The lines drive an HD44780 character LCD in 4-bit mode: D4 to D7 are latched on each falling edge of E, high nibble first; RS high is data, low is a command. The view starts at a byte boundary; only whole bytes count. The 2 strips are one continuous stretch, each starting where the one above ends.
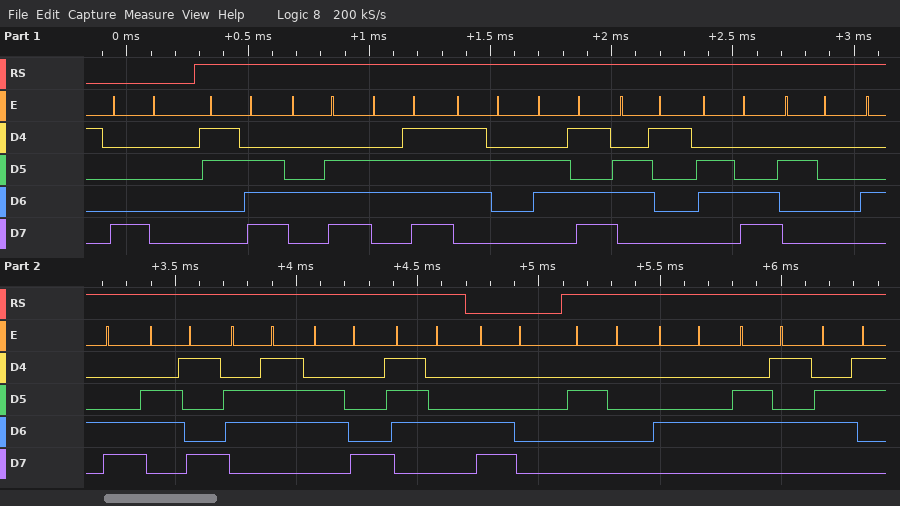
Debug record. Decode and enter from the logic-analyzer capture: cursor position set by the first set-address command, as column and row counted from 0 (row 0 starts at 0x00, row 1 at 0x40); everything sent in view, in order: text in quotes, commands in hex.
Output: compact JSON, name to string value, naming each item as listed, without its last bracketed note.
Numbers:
{"cursor position set by the first set-address command, as column and row counted from 0": "column 0, row 0", "everything sent in view, in order: text in quotes, commands in hex": "0x80 \">Normal Light\" 0xC0 \" Dec\""}
